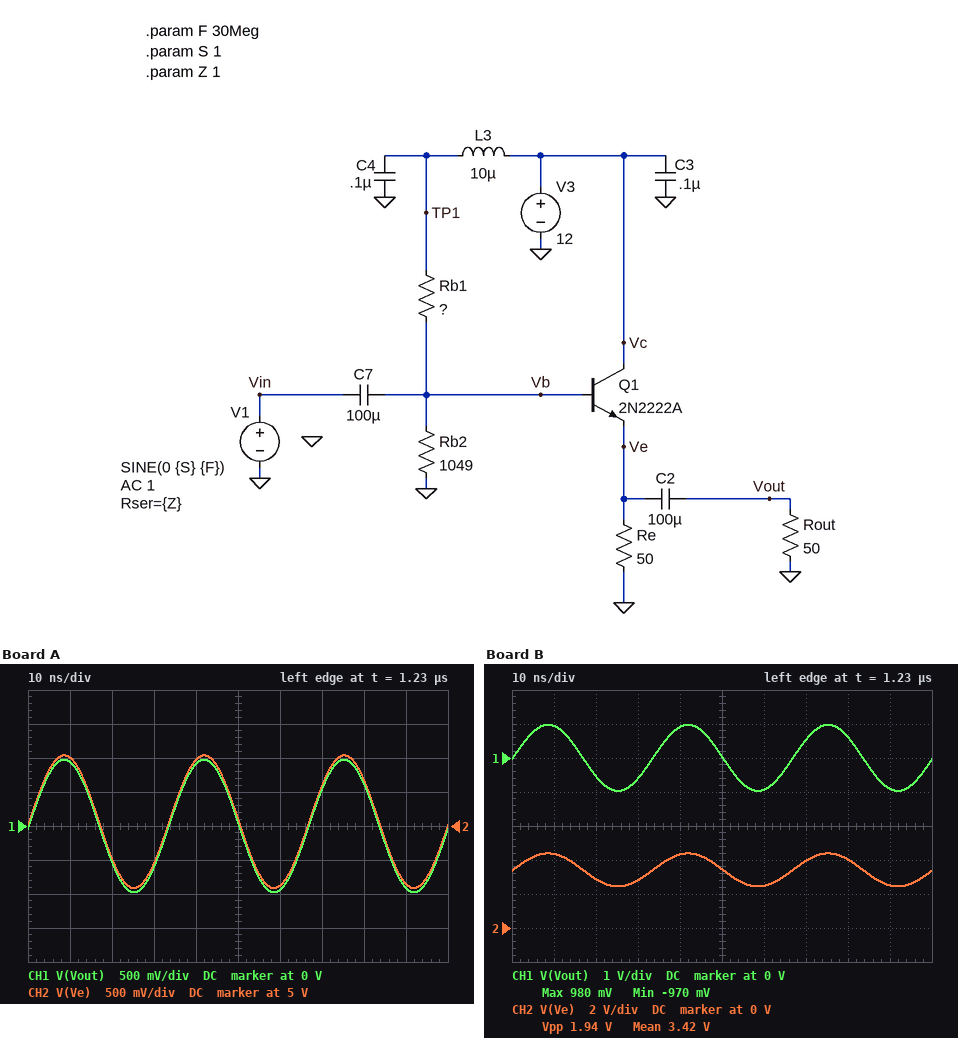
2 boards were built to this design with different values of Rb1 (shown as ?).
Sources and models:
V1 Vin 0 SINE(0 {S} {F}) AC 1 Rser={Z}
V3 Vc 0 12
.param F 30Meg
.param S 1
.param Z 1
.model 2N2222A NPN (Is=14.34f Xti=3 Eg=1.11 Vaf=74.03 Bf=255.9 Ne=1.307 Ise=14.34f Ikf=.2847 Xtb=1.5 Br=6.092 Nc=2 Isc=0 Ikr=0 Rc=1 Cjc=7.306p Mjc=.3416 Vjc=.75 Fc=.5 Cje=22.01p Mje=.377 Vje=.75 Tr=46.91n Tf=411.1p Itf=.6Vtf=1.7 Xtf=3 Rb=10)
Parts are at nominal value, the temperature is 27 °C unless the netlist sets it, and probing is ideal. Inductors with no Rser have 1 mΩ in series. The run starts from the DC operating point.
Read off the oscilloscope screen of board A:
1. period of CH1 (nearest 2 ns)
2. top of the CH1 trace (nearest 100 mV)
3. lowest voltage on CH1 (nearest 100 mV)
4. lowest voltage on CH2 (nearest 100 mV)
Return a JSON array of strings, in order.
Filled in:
["34 ns", "1.0 V", "-1.0 V", "4.1 V"]
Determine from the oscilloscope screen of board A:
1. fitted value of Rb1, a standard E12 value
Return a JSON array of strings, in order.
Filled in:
["1 kΩ"]
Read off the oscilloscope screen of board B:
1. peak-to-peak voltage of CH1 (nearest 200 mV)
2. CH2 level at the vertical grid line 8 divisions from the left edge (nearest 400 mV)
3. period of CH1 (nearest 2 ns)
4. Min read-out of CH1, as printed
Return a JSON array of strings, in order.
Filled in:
["2.0 V", "4.0 V", "34 ns", "-970 mV"]
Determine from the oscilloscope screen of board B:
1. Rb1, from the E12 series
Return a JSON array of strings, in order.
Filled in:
["1.8 kΩ"]
